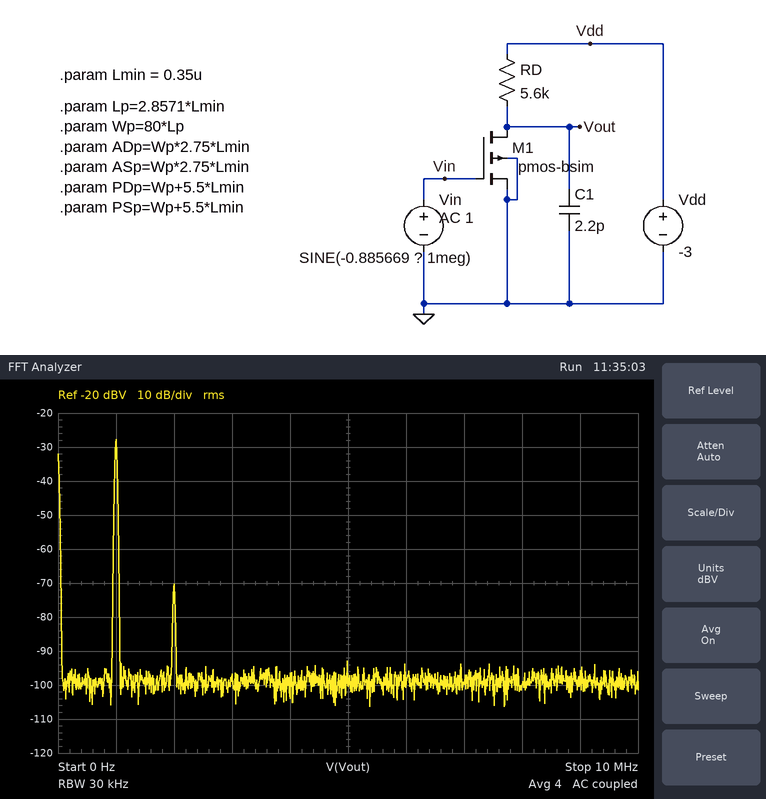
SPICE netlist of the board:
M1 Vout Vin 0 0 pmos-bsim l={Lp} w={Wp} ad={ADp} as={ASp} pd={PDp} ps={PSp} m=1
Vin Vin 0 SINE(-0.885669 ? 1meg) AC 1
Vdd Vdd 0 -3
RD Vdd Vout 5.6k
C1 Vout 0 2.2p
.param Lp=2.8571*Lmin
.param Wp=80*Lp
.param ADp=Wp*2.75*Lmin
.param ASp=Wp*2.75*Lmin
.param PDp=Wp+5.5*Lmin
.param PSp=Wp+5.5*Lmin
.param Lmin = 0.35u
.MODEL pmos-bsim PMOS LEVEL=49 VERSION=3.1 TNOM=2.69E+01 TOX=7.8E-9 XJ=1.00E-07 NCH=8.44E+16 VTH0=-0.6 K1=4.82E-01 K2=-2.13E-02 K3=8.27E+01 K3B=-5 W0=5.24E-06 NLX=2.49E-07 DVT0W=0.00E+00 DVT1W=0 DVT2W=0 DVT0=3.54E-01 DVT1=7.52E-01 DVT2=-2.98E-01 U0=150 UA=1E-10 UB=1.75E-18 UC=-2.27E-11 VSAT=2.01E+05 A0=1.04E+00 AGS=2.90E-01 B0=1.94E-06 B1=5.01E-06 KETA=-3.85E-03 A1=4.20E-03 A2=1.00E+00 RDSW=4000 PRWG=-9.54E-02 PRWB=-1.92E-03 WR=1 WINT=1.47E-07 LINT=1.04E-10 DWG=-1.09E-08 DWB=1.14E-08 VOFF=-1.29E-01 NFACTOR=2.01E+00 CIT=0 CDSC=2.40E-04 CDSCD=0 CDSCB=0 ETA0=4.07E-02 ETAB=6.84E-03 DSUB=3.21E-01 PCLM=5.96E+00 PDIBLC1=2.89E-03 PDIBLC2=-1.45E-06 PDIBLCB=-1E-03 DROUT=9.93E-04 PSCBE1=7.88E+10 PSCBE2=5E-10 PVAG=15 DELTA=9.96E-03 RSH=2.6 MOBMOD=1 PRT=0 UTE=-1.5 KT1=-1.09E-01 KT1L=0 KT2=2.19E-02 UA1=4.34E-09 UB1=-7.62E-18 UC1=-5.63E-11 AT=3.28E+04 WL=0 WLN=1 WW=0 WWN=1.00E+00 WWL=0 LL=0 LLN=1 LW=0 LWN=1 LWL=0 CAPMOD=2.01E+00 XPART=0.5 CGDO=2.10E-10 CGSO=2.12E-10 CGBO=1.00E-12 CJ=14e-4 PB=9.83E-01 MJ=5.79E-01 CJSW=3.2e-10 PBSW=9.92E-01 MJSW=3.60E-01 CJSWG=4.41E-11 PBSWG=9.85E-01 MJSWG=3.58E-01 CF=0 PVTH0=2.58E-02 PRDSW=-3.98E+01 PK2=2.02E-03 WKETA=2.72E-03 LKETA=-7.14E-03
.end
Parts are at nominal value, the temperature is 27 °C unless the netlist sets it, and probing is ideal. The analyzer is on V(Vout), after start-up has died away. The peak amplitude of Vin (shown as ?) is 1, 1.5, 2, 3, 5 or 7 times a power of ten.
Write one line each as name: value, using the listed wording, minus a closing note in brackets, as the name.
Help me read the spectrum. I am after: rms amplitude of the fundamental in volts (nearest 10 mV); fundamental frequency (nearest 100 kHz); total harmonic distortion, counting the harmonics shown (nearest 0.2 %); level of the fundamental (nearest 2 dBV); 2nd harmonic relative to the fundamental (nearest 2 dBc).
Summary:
rms amplitude of the fundamental in volts: 40 mV
fundamental frequency: 1.0 MHz
total harmonic distortion, counting the harmonics shown: 0.8 %
level of the fundamental: -28 dBV
2nd harmonic relative to the fundamental: -42 dBc
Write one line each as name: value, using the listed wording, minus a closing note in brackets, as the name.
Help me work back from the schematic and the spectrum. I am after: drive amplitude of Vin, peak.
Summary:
drive amplitude of Vin, peak: 10 mV
